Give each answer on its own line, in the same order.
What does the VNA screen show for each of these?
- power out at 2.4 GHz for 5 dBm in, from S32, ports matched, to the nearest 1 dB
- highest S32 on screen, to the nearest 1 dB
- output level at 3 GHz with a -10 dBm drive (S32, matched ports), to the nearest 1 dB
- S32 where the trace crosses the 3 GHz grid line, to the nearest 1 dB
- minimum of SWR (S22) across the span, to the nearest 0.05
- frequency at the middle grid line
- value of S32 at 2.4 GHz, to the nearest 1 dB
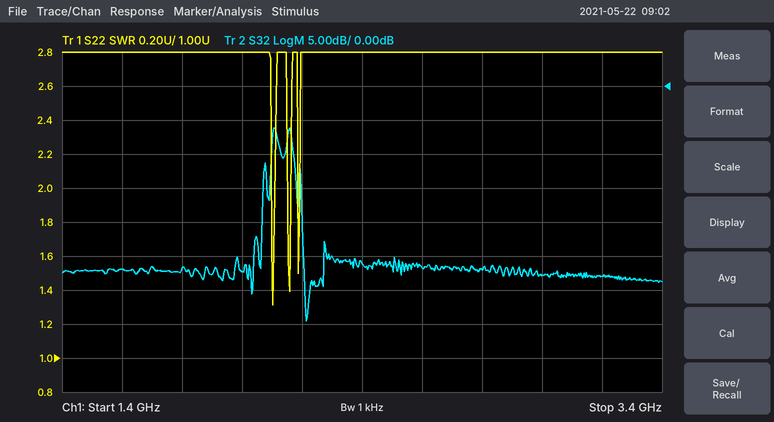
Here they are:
-21 dBm
-6 dB
-38 dBm
-28 dB
1.30
2.4 GHz
-26 dB
